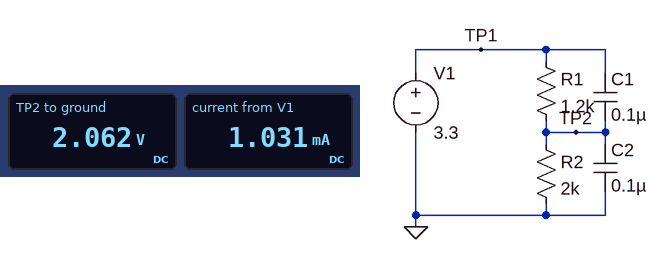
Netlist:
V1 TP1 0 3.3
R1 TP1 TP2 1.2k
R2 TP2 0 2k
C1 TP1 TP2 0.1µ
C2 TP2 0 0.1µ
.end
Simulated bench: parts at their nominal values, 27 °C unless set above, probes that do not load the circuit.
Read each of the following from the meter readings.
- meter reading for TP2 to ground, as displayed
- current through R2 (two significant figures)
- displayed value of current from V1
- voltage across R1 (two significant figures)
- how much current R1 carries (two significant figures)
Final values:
2.062 V
1.0 mA
1.031 mA
1.2 V
1.0 mA
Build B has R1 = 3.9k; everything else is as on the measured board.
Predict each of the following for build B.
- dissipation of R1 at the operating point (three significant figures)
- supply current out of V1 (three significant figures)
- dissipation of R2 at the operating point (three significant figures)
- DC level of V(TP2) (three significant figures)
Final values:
1.22 mW
559 µA
626 µW
1.12 V
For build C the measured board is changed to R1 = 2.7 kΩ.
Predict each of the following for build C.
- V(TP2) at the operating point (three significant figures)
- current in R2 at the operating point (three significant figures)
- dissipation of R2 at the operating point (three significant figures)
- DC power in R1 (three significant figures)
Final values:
1.40 V
702 µA
986 µW
1.33 mW
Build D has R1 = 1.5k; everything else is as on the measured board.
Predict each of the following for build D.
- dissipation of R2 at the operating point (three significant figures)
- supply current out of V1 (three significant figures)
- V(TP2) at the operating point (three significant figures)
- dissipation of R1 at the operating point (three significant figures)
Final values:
1.78 mW
943 µA
1.89 V
1.33 mW
